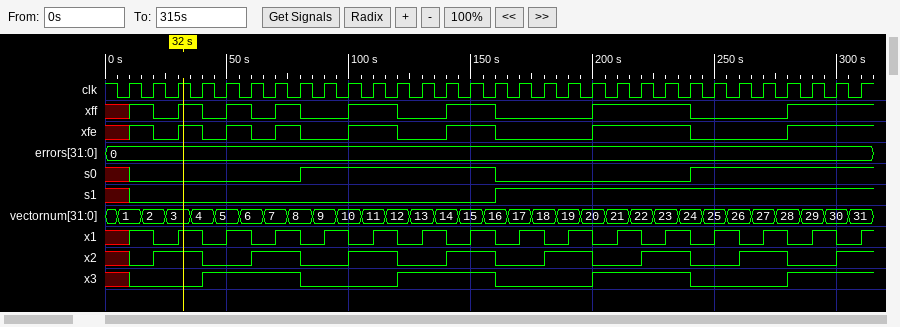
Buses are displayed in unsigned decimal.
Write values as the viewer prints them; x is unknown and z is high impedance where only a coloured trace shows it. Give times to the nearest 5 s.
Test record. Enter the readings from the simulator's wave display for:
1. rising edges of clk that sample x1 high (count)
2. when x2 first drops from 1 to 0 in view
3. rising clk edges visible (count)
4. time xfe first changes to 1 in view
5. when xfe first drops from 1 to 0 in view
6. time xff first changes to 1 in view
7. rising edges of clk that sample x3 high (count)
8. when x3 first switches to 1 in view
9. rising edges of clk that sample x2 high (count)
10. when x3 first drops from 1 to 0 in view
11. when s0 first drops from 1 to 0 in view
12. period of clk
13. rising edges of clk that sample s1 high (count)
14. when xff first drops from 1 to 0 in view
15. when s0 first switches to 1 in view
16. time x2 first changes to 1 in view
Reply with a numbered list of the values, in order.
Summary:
1. 15
2. 40 s
3. 31
4. 10 s
5. 20 s
6. 10 s
7. 15
8. 40 s
9. 15
10. 80 s
11. 160 s
12. 10 s
13. 15
14. 20 s
15. 80 s
16. 20 s
